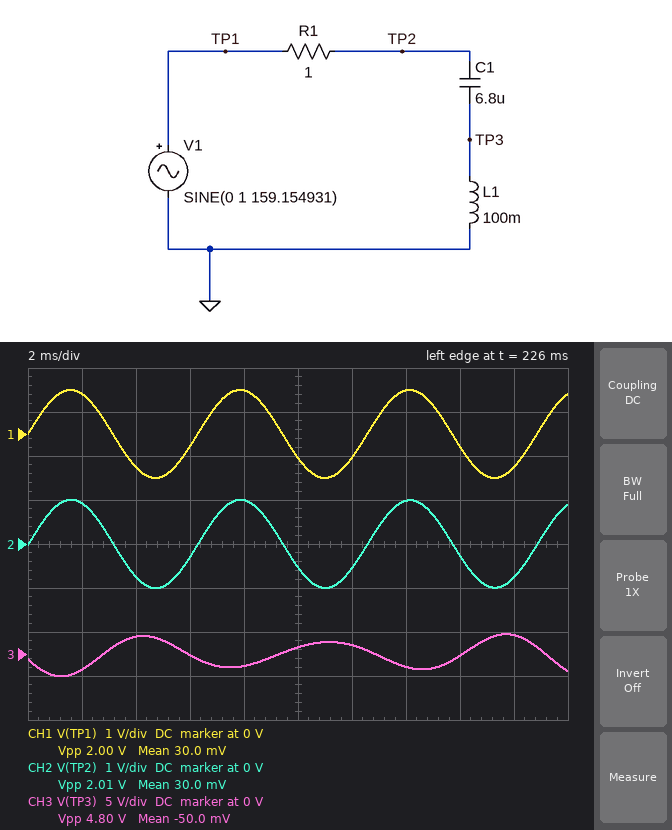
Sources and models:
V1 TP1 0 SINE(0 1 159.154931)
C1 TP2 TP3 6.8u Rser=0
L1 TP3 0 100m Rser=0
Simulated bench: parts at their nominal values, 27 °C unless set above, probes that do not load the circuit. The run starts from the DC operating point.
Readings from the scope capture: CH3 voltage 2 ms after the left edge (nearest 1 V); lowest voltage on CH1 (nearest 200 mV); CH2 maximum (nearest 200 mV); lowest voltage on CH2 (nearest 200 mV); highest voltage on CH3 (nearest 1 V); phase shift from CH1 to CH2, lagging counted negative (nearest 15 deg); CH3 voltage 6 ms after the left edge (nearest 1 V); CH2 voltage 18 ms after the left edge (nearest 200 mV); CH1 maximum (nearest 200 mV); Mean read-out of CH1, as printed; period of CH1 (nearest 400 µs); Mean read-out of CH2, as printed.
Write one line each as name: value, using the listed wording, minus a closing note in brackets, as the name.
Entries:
CH3 voltage 2 ms after the left edge: -2 V
lowest voltage on CH1: -1.0 V
CH2 maximum: 1.0 V
lowest voltage on CH2: -1.0 V
highest voltage on CH3: 2 V
phase shift from CH1 to CH2, lagging counted negative: 0 deg
CH3 voltage 6 ms after the left edge: 0 V
CH2 voltage 18 ms after the left edge: -800 mV
CH1 maximum: 1.0 V
Mean read-out of CH1, as printed: 30.0 mV
period of CH1: 6.4 ms
Mean read-out of CH2, as printed: 30.0 mV
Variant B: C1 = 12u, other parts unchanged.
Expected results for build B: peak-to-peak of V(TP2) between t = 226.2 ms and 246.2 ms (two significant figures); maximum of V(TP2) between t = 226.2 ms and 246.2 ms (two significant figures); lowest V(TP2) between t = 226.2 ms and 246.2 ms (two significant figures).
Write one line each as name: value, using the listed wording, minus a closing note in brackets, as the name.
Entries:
peak-to-peak of V(TP2) between t = 226.2 ms and 246.2 ms: 2.0 V
maximum of V(TP2) between t = 226.2 ms and 246.2 ms: 980 mV
lowest V(TP2) between t = 226.2 ms and 246.2 ms: -990 mV
